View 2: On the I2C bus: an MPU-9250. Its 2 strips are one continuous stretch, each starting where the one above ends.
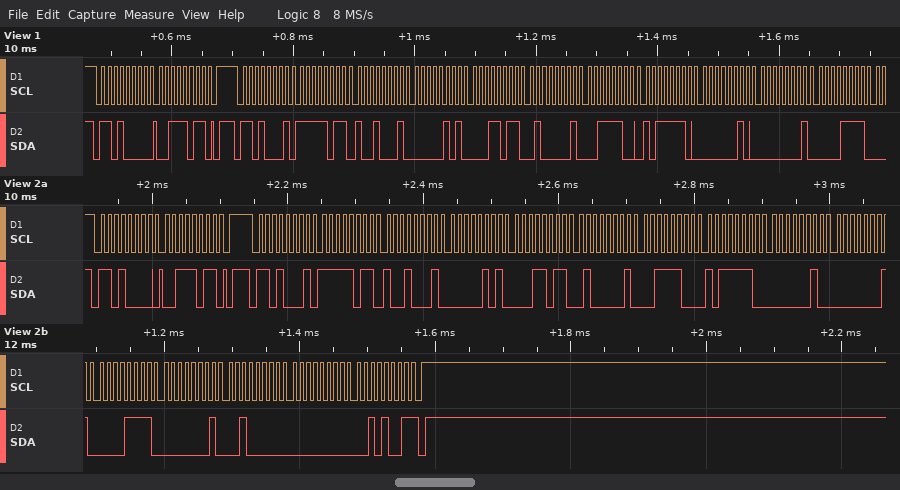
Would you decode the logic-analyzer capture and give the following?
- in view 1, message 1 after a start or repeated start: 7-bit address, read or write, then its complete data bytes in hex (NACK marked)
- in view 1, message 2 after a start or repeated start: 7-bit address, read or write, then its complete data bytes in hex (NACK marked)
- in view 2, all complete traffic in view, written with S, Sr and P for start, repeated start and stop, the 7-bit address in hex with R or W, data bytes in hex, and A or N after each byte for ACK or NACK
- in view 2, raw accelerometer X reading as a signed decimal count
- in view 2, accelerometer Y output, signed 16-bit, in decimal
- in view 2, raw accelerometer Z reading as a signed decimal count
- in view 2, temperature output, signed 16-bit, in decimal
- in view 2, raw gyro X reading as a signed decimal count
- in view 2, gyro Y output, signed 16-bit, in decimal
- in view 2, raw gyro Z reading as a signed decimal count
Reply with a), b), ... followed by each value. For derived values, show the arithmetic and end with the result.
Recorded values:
a) 0x68 write: 3B
b) 0x68 read: FB 91 05 1B 41 3C BE 02 01 0F
c) S 68W A 3B A P S 68R A FB A 91 A 05 A 1B A 41 A 3C A BE A 02 A 01 A 0F A 01 A 20 A 00 A 29 N P
d) 0xFB91 = -1135
e) 0x051B = 1307
f) 0x413C = 16700
g) 0xBE02 = -16894
h) 0x010F = 271
i) 0x0120 = 288
j) 0x0029 = 41
